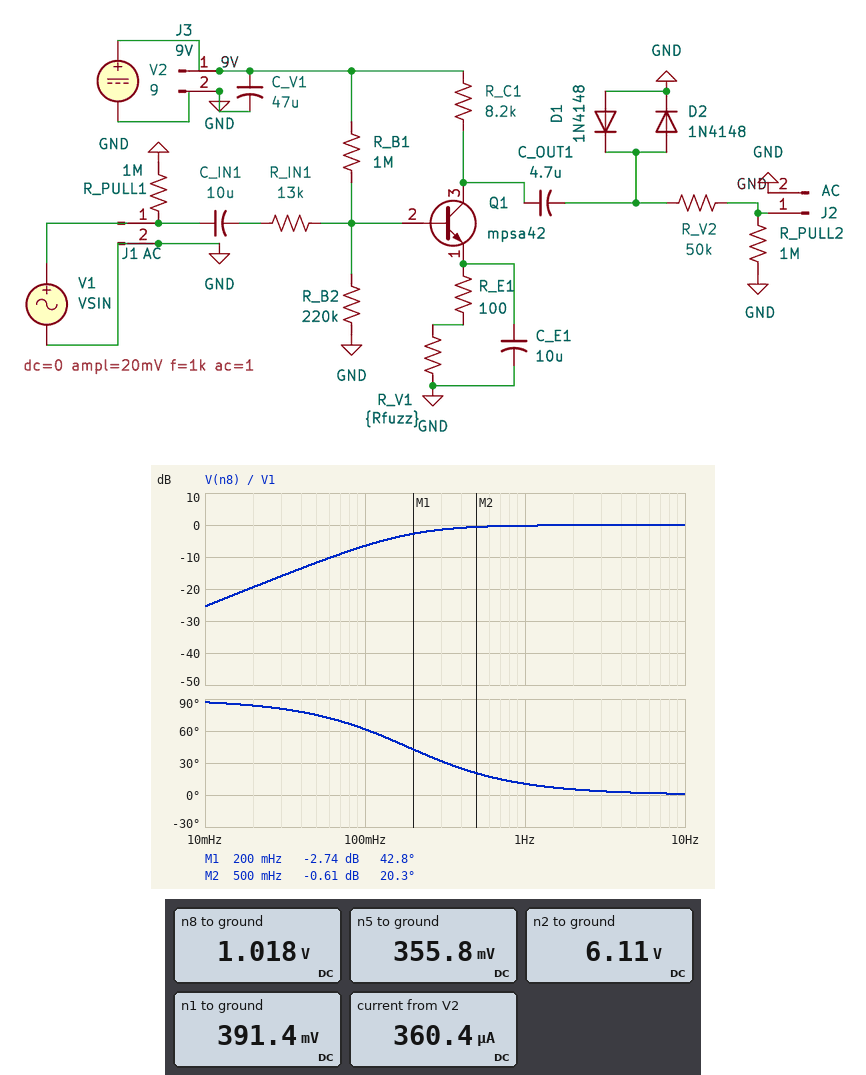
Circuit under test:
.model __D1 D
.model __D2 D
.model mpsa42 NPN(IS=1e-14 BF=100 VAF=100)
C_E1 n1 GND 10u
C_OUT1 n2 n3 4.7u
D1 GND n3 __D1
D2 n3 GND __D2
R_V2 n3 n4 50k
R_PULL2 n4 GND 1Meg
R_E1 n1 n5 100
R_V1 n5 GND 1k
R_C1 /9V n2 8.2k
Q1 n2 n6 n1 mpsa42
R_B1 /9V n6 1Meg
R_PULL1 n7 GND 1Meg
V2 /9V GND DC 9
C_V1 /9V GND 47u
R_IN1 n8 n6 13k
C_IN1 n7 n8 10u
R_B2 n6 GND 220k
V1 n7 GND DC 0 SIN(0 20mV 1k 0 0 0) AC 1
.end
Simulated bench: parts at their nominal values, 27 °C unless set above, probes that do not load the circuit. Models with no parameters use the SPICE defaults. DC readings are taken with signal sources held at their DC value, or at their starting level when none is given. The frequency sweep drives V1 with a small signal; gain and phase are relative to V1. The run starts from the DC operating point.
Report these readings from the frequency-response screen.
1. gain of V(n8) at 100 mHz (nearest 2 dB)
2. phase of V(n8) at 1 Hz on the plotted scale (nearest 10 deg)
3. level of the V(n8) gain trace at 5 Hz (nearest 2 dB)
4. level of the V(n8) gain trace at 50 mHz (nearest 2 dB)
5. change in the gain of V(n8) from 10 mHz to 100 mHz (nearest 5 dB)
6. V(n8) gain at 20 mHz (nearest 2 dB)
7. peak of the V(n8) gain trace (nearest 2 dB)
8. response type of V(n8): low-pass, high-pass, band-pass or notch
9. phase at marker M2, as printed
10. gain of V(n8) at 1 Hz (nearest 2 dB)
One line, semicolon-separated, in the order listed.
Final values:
-6 dB; 10 deg; 0 dB; -12 dB; 20 dB; -20 dB; 0 dB; high-pass; 20.3 deg; 0 dB
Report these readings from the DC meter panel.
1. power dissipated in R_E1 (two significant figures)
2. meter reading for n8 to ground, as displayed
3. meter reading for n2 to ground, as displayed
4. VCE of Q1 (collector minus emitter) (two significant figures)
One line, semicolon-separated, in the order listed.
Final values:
13 µW; 1.018 V; 6.11 V; 5.7 V
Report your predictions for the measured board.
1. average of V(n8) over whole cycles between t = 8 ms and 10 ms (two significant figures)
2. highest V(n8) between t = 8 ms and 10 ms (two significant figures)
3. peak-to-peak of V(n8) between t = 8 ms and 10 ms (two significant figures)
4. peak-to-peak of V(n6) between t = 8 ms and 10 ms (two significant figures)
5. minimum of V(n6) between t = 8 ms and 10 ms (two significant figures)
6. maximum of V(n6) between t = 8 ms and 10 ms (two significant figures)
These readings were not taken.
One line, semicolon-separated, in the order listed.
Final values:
1.0 V; 1.0 V; 40 mV; 15 mV; 1.0 V; 1.0 V
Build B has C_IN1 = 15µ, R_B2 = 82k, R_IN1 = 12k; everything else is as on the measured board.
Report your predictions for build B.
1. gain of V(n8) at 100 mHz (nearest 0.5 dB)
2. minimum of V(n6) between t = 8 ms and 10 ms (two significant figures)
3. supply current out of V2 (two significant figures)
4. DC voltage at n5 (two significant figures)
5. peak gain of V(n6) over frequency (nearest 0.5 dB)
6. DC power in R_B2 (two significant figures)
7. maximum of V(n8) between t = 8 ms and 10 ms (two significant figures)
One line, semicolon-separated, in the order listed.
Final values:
-5.5 dB; 630 mV; 65 µA; 57 mV; -2.0 dB; 5.0 µW; 660 mV
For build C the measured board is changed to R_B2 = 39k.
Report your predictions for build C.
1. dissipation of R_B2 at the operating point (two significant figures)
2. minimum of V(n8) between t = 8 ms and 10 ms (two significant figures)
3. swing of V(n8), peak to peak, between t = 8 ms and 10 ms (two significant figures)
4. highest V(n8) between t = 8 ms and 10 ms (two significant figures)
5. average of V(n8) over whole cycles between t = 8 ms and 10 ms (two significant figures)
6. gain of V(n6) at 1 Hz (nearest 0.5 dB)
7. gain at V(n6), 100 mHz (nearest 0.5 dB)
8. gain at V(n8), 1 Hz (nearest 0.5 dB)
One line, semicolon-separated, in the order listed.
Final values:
2.9 µW; 320 mV; 40 mV; 360 mV; 340 mV; -3.0 dB; -13.0 dB; -0.5 dB
